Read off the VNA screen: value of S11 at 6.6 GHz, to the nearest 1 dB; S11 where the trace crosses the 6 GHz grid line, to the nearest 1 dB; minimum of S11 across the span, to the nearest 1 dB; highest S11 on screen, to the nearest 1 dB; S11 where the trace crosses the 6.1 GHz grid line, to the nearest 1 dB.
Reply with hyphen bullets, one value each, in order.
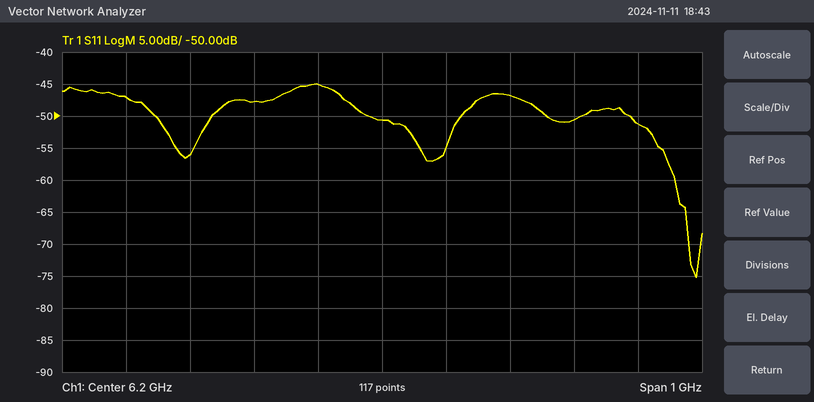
- -51 dB
- -48 dB
- -75 dB
- -45 dB
- -45 dB
